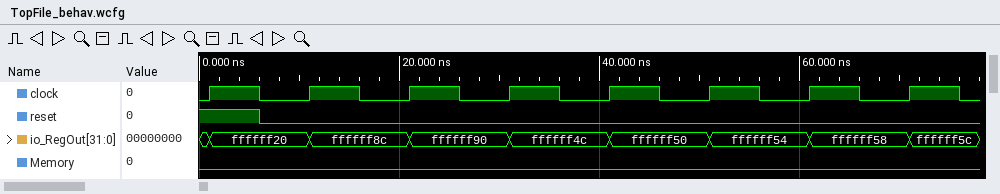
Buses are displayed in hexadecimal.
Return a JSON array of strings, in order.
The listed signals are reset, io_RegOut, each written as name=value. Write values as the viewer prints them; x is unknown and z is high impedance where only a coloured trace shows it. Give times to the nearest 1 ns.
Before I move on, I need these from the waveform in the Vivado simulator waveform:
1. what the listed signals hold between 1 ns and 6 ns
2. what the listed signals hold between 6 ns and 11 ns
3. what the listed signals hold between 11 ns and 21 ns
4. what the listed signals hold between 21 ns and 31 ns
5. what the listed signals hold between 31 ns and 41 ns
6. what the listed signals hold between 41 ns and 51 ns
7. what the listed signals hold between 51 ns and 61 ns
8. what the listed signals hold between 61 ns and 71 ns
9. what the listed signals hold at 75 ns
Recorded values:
["reset=1, io_RegOut=ffffff20", "reset=0, io_RegOut=ffffff20", "reset=0, io_RegOut=ffffff8c", "reset=0, io_RegOut=ffffff90", "reset=0, io_RegOut=ffffff4c", "reset=0, io_RegOut=ffffff50", "reset=0, io_RegOut=ffffff54", "reset=0, io_RegOut=ffffff58", "reset=0, io_RegOut=ffffff5c"]
